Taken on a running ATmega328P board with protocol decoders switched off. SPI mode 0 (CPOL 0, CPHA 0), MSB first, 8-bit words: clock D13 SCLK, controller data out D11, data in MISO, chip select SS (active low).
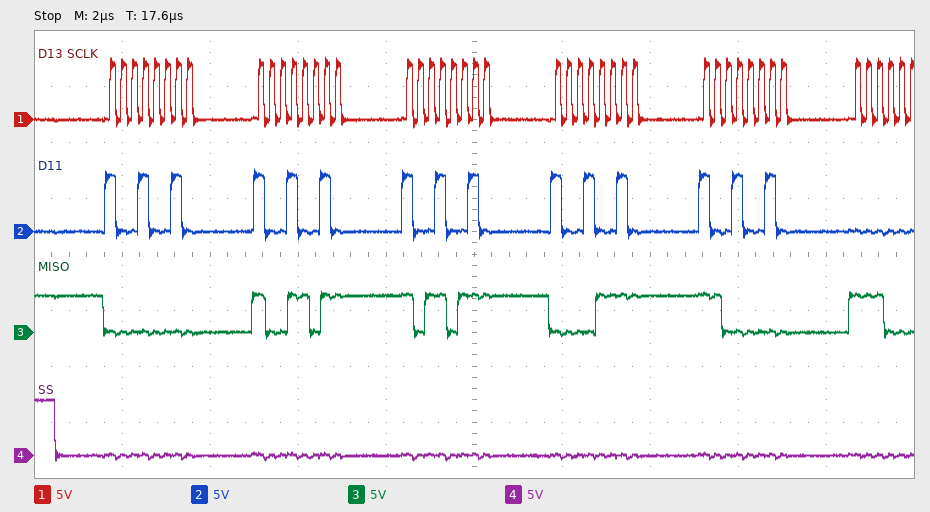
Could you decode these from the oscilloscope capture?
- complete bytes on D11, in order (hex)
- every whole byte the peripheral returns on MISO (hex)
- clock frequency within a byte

92 92 92 92 92
00 9B B7 0F C0
4 MHz
